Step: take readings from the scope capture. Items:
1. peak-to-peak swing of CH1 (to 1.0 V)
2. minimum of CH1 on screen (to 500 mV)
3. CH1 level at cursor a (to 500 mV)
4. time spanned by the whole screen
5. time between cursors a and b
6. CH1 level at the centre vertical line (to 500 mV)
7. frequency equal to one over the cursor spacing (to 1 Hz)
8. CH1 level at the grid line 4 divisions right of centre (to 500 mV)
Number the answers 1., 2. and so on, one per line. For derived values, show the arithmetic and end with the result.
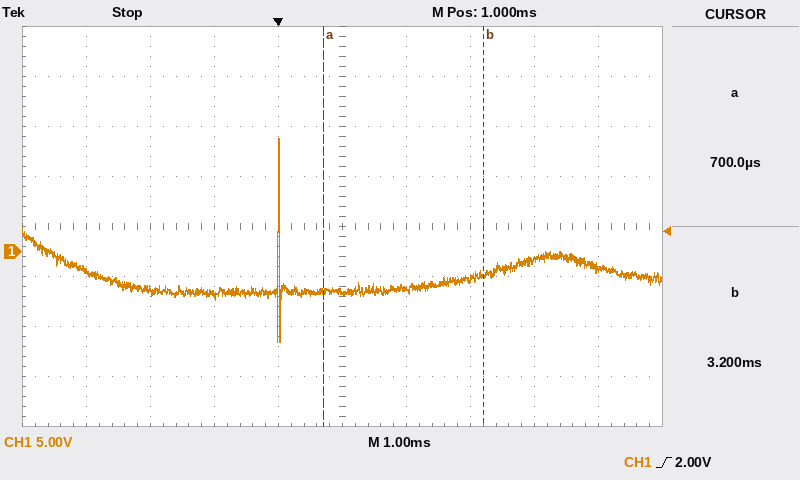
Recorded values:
1. 20.0 V
2. -9.0 V
3. -4.0 V
4. 10 ms
5. 3.2 ms − (700 µs) = 2.5 ms
6. -4.0 V
7. 1 / 2.5 ms ≈ 400 Hz
8. -1.5 V
